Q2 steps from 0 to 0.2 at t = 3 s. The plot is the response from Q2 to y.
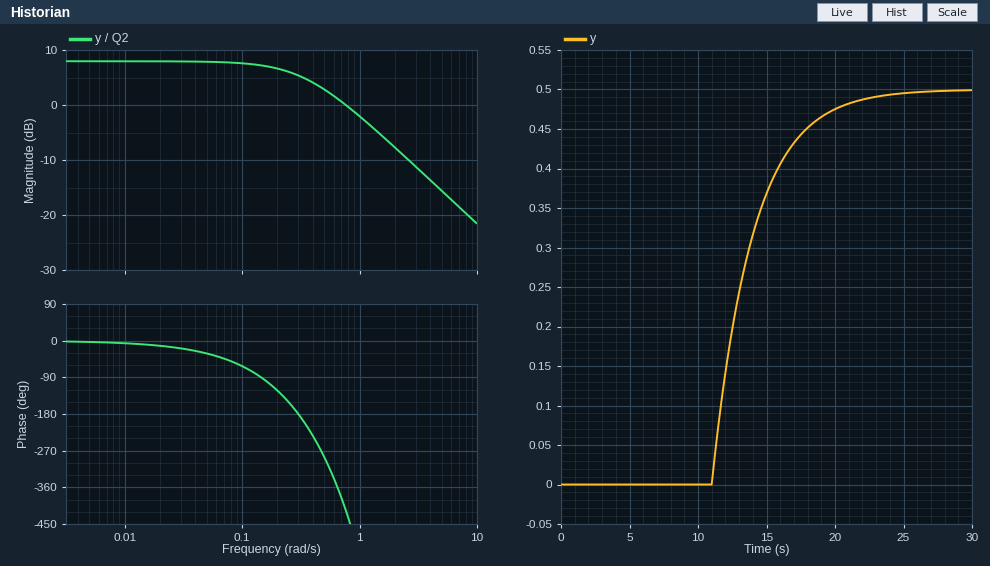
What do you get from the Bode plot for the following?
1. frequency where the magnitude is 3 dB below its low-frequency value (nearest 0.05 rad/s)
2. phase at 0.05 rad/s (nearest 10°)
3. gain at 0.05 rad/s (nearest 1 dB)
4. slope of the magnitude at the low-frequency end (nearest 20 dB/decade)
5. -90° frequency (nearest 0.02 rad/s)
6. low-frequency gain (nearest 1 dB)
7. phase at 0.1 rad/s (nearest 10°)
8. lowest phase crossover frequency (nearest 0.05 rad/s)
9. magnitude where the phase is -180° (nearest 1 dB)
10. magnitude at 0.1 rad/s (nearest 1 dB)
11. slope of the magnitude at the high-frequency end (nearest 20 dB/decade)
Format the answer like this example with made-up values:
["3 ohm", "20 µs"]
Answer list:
["0.35 rad/s", "-30°", "8 dB", "0 dB/decade", "0.14 rad/s", "8 dB", "-60°", "0.30 rad/s", "5 dB", "8 dB", "-20 dB/decade"]
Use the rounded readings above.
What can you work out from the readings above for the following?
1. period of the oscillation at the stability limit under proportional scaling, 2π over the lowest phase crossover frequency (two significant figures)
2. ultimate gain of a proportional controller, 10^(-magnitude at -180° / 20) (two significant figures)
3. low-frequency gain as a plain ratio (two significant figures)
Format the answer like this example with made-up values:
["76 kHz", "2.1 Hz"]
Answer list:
["21 s", "0.56", "2.5"]
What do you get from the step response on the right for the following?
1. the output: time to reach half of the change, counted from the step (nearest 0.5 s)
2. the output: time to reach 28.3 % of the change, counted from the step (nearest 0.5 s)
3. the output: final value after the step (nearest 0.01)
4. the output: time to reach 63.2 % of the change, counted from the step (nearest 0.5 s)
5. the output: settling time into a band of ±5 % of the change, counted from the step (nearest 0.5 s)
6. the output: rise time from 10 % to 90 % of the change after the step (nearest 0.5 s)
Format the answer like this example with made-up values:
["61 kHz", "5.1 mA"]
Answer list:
["10.0 s", "9.0 s", "0.50", "11.0 s", "17.0 s", "6.5 s"]
